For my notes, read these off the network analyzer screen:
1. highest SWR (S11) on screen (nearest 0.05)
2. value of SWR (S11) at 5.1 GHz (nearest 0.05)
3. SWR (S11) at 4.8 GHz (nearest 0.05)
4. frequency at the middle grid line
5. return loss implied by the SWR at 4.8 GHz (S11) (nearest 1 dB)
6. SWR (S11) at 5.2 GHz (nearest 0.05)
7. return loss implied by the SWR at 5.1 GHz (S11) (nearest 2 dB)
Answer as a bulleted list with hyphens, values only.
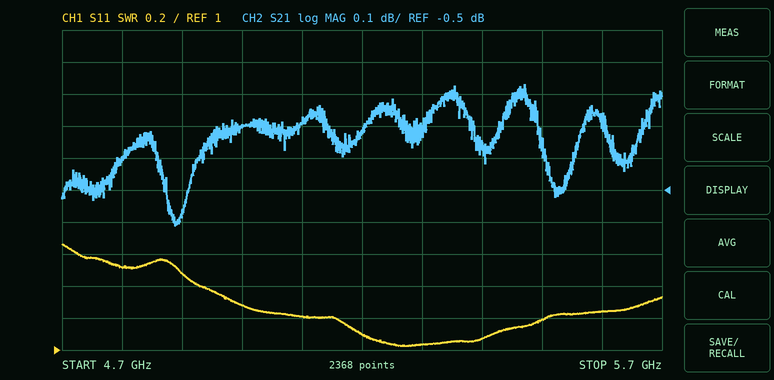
- 1.65
- 1.20
- 1.50
- 5.2 GHz
- 14 dB
- 1.10
- 20 dB
